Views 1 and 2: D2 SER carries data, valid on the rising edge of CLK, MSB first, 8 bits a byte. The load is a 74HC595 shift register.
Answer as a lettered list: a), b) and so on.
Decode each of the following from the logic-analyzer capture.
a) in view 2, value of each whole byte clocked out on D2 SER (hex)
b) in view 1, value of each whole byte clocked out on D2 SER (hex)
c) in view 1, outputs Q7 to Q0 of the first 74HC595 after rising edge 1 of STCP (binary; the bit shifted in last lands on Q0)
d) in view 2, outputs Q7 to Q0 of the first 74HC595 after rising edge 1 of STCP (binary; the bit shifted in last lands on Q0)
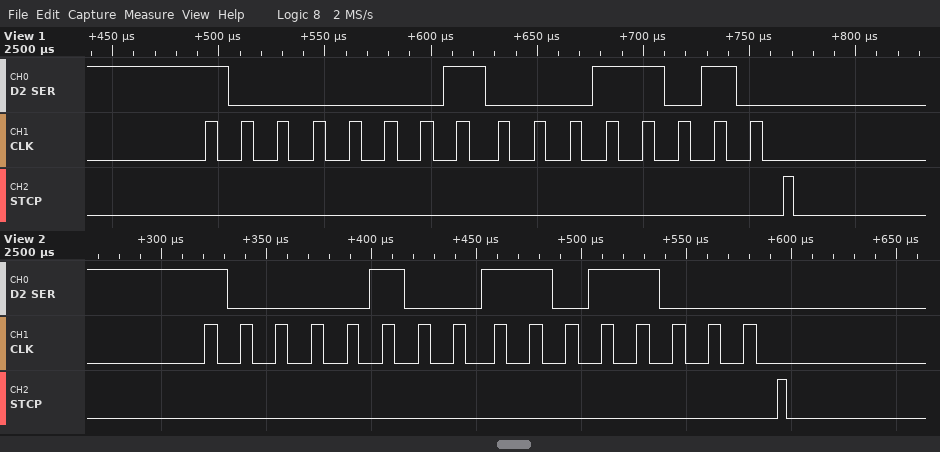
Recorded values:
a) 0x84 0xD8
b) 0x81 0x1A
c) 00011010
d) 11011000
